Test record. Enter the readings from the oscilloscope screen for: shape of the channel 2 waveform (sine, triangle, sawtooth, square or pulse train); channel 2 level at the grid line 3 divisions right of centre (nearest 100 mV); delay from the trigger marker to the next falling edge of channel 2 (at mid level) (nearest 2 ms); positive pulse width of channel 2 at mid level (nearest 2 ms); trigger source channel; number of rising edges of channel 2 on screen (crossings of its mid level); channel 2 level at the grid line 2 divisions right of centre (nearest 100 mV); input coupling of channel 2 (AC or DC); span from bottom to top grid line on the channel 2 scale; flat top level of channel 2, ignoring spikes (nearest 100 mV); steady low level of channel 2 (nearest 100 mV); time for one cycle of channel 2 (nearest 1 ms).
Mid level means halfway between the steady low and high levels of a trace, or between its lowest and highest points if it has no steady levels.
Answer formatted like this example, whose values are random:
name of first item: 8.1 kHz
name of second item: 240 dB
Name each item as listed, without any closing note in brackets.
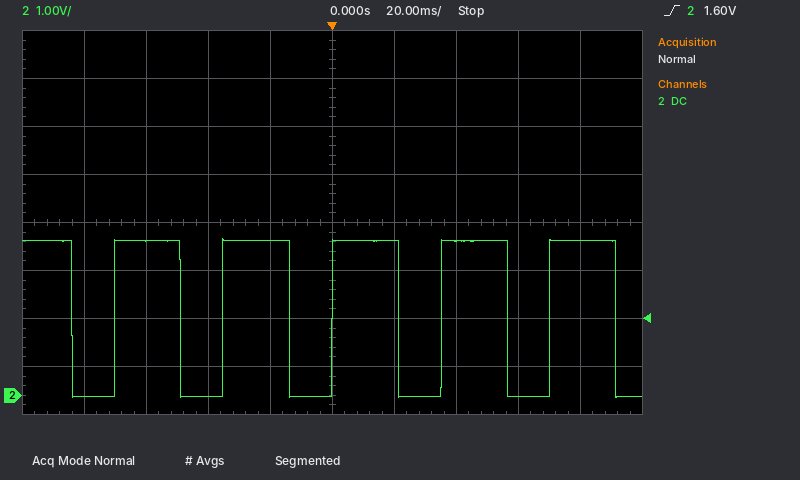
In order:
shape of the channel 2 waveform: pulse train
channel 2 level at the grid line 3 divisions right of centre: 0.0 V
delay from the trigger marker to the next falling edge of channel 2 (at mid level): 22 ms
positive pulse width of channel 2 at mid level: 22 ms
trigger source channel: channel 2
number of rising edges of channel 2 on screen: 5
channel 2 level at the grid line 2 divisions right of centre: 3.2 V
input coupling of channel 2: DC
span from bottom to top grid line on the channel 2 scale: 8 V
flat top level of channel 2, ignoring spikes: 3.2 V
steady low level of channel 2: 0.0 V
time for one cycle of channel 2: 35 ms
